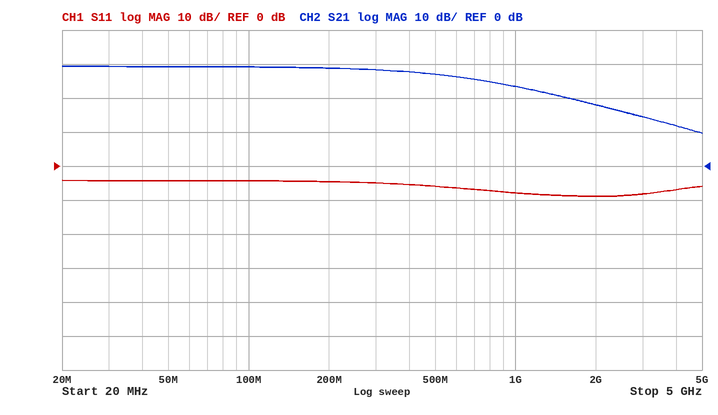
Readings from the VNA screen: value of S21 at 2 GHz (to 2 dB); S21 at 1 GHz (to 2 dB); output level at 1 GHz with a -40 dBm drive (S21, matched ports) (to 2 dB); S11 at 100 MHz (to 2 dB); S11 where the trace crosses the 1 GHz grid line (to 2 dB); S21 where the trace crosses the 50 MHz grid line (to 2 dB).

18 dB
24 dB
-16 dBm
-4 dB
-8 dB
30 dB
